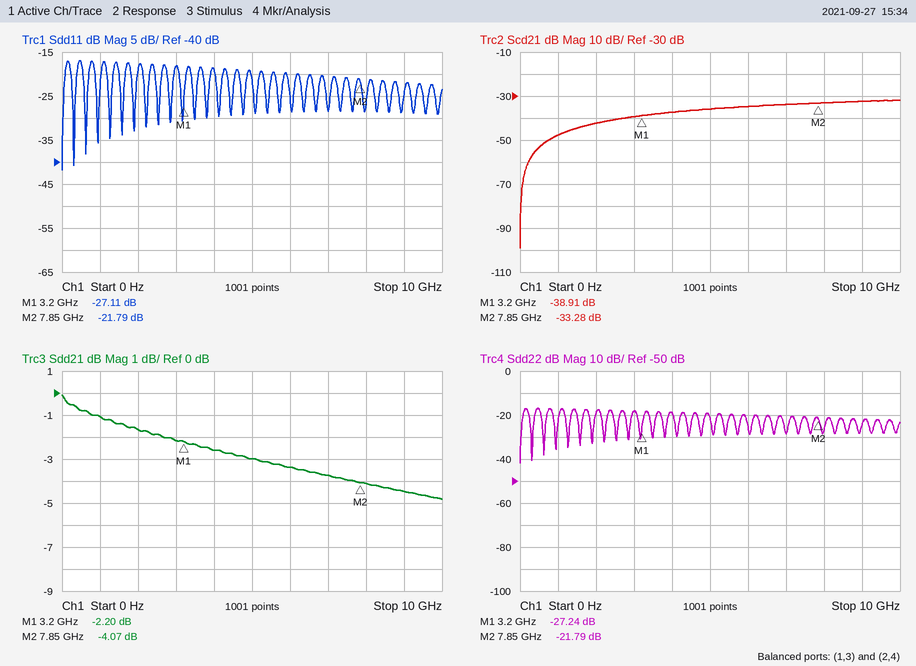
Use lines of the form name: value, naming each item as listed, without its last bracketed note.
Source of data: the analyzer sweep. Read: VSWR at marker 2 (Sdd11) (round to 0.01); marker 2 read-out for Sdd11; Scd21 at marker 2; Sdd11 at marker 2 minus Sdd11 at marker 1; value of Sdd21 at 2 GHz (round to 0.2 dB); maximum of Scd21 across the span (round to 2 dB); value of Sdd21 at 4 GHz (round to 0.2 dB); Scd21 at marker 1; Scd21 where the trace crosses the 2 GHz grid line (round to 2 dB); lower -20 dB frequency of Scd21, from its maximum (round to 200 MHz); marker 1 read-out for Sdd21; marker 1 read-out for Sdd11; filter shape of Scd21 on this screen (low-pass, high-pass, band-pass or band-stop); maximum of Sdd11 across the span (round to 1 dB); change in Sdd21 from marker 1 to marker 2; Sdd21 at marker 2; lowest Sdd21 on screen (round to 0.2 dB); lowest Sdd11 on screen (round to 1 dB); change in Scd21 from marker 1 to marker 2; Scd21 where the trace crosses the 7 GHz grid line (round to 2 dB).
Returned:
VSWR at marker 2 (Sdd11): 1.18
marker 2 read-out for Sdd11: -21.79 dB
Scd21 at marker 2: -33.28 dB
Sdd11 at marker 2 minus Sdd11 at marker 1: 5.32 dB
value of Sdd21 at 2 GHz: -1.6 dB
maximum of Scd21 across the span: -32 dB
value of Sdd21 at 4 GHz: -2.6 dB
Scd21 at marker 1: -38.91 dB
Scd21 where the trace crosses the 2 GHz grid line: -42 dB
lower -20 dB frequency of Scd21, from its maximum: 600 MHz
marker 1 read-out for Sdd21: -2.20 dB
marker 1 read-out for Sdd11: -27.11 dB
filter shape of Scd21 on this screen: high-pass
maximum of Sdd11 across the span: -17 dB
change in Sdd21 from marker 1 to marker 2: -1.87 dB
Sdd21 at marker 2: -4.07 dB
lowest Sdd21 on screen: -4.8 dB
lowest Sdd11 on screen: -42 dB
change in Scd21 from marker 1 to marker 2: 5.63 dB
Scd21 where the trace crosses the 7 GHz grid line: -34 dB
